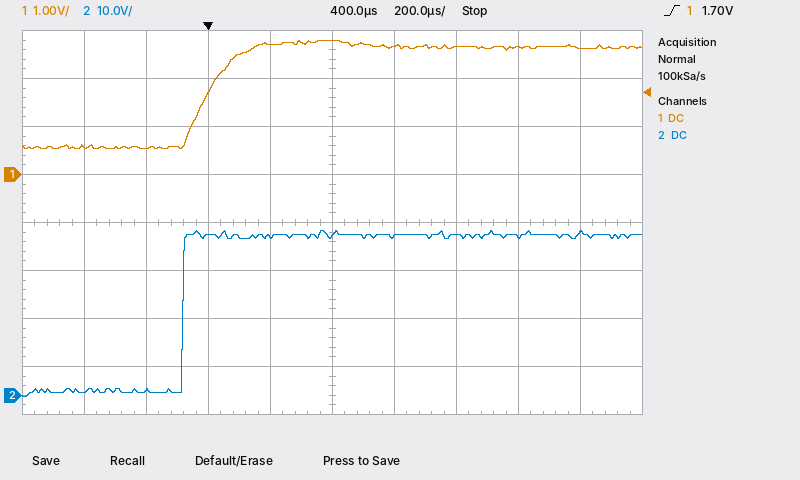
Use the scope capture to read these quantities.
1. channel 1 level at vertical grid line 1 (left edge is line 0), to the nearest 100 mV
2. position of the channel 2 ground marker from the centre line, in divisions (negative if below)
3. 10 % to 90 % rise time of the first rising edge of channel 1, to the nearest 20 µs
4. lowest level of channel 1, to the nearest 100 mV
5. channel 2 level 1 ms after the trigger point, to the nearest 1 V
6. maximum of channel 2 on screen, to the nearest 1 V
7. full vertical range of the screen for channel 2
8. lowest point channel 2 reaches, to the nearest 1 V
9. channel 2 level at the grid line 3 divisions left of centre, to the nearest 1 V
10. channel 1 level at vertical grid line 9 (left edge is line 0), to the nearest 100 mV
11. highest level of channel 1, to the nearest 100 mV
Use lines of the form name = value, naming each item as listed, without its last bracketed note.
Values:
channel 1 level at vertical grid line 1 (left edge is line 0), to the nearest 100 mV = 600 mV
position of the channel 2 ground marker from the centre line, in divisions = -3.6 div
10 % to 90 % rise time of the first rising edge of channel 1, to the nearest 20 µs = 160 µs
lowest level of channel 1, to the nearest 100 mV = 500 mV
channel 2 level 1 ms after the trigger point, to the nearest 1 V = 33 V
maximum of channel 2 on screen, to the nearest 1 V = 34 V
full vertical range of the screen for channel 2 = 80 V
lowest point channel 2 reaches, to the nearest 1 V = 0 V
channel 2 level at the grid line 3 divisions left of centre, to the nearest 1 V = 1 V
channel 1 level at vertical grid line 9 (left edge is line 0), to the nearest 100 mV = 2.6 V
highest level of channel 1, to the nearest 100 mV = 2.8 V
